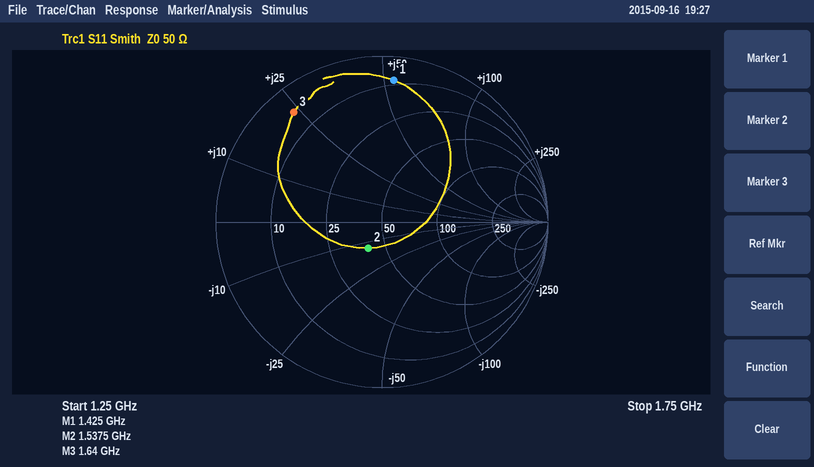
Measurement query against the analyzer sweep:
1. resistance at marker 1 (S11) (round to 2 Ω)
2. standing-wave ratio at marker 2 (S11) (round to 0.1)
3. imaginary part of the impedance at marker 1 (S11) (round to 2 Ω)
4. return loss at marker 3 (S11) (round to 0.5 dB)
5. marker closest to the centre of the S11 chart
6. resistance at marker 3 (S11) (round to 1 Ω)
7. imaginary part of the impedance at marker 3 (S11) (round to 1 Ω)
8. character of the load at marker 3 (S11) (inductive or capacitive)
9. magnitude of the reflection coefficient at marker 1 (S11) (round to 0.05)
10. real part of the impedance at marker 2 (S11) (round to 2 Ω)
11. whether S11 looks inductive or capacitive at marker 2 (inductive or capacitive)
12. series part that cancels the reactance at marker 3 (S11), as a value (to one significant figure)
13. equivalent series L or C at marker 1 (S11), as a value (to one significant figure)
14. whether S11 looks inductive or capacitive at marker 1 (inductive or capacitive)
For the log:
8 Ω
1.4
+54 Ω
1.5 dB
marker 2
5 Ω
+24 Ω
inductive
0.85
40 Ω
capacitive
4 pF
6 nH
inductive
